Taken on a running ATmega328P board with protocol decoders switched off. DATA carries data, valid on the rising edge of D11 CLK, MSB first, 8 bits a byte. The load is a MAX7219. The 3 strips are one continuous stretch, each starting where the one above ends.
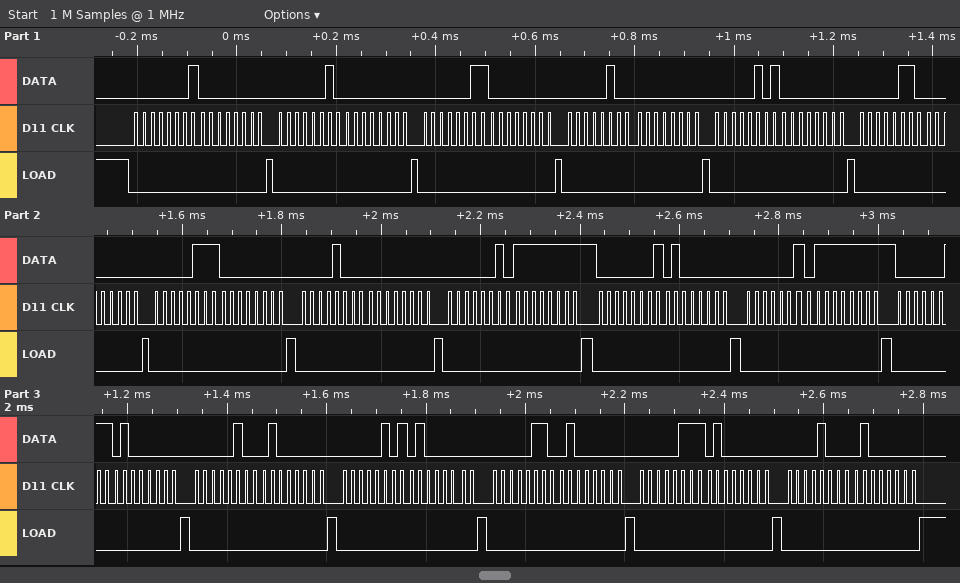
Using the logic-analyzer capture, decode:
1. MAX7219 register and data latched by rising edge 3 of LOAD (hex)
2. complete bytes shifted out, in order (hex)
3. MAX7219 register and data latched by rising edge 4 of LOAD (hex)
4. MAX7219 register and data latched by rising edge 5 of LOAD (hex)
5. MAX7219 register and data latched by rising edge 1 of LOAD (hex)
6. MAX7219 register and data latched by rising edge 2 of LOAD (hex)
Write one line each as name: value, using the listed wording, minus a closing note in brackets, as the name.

MAX7219 register and data latched by rising edge 3 of LOAD: register 0x3, data 0x00
complete bytes shifted out, in order: 0x01 0x00 0x02 0x00 0x03 0x00 0x04 0x00 0x05 0x00 0x06 0x00 0x07 0x00 0x08 0x00 0x02 0xFF 0x01 0x40 0x02 0xFF 0x03 0x40 0x04 0x40 0x05 0x40 0x06 0x40 0x07 0x40 0x08 0x40
MAX7219 register and data latched by rising edge 4 of LOAD: register 0x4, data 0x00
MAX7219 register and data latched by rising edge 5 of LOAD: register 0x5, data 0x00
MAX7219 register and data latched by rising edge 1 of LOAD: register 0x1, data 0x00
MAX7219 register and data latched by rising edge 2 of LOAD: register 0x2, data 0x00
